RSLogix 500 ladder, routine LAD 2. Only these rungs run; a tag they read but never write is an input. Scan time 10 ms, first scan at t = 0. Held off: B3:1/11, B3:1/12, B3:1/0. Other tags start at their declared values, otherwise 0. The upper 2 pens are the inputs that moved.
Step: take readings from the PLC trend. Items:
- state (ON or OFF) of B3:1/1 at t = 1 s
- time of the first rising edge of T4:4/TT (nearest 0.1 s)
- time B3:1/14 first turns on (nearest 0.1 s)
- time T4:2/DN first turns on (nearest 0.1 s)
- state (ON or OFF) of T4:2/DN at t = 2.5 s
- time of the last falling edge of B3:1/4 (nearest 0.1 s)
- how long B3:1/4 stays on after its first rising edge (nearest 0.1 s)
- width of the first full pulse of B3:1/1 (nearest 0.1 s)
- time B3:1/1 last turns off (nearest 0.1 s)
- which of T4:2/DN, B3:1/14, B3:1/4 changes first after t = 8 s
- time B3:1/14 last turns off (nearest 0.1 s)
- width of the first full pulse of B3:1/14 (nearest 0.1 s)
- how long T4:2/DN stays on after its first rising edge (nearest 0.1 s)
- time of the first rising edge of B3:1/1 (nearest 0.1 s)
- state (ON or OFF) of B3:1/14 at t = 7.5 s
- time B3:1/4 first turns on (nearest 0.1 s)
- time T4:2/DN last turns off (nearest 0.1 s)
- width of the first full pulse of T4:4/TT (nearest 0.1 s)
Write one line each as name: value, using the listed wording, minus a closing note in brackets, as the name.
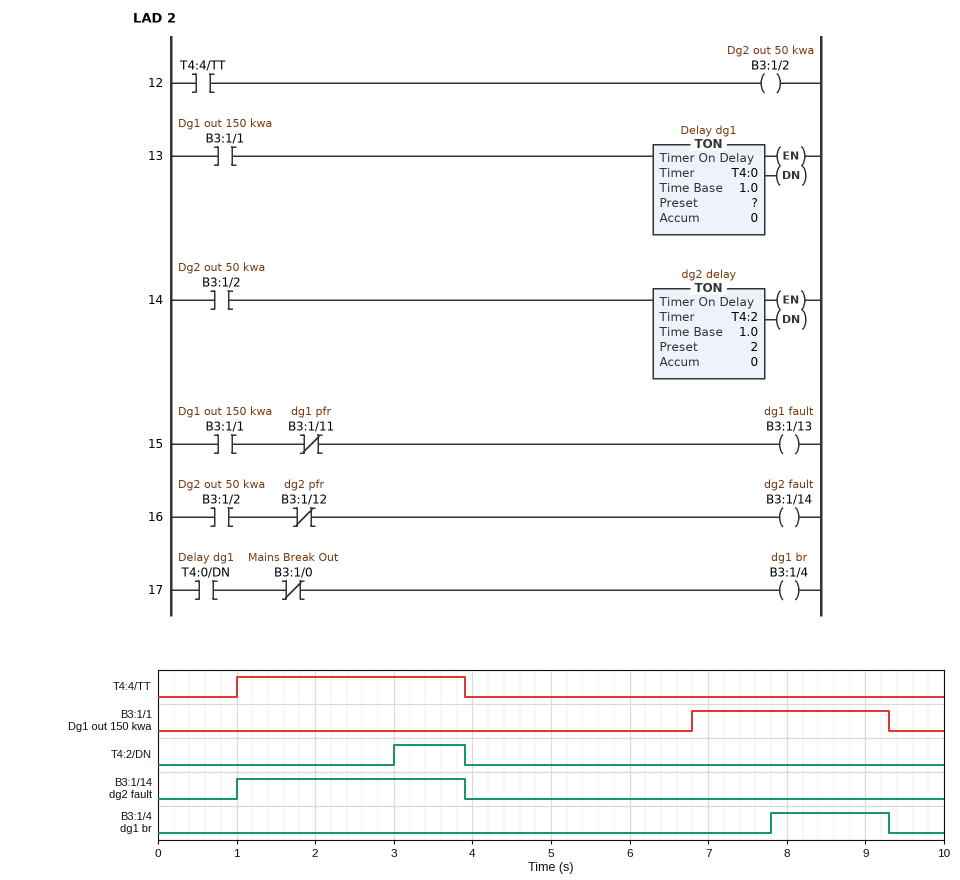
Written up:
state (ON or OFF) of B3:1/1 at t = 1 s: OFF
time of the first rising edge of T4:4/TT: 1.0 s
time B3:1/14 first turns on: 1.0 s
time T4:2/DN first turns on: 3.0 s
state (ON or OFF) of T4:2/DN at t = 2.5 s: OFF
time of the last falling edge of B3:1/4: 9.3 s
how long B3:1/4 stays on after its first rising edge: 1.5 s
width of the first full pulse of B3:1/1: 2.5 s
time B3:1/1 last turns off: 9.3 s
which of T4:2/DN, B3:1/14, B3:1/4 changes first after t = 8 s: B3:1/4
time B3:1/14 last turns off: 3.9 s
width of the first full pulse of B3:1/14: 2.9 s
how long T4:2/DN stays on after its first rising edge: 0.9 s
time of the first rising edge of B3:1/1: 6.8 s
state (ON or OFF) of B3:1/14 at t = 7.5 s: OFF
time B3:1/4 first turns on: 7.8 s
time T4:2/DN last turns off: 3.9 s
width of the first full pulse of T4:4/TT: 2.9 s
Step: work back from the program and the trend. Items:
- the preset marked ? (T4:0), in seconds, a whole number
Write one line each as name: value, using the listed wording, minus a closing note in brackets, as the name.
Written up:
the preset marked ? (T4:0), in seconds, a whole number: 1 s
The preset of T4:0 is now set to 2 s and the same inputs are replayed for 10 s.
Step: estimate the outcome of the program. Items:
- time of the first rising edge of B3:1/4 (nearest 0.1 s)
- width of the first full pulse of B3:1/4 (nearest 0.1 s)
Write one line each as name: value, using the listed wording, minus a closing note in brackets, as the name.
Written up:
time of the first rising edge of B3:1/4: 8.8 s
width of the first full pulse of B3:1/4: 0.5 s
